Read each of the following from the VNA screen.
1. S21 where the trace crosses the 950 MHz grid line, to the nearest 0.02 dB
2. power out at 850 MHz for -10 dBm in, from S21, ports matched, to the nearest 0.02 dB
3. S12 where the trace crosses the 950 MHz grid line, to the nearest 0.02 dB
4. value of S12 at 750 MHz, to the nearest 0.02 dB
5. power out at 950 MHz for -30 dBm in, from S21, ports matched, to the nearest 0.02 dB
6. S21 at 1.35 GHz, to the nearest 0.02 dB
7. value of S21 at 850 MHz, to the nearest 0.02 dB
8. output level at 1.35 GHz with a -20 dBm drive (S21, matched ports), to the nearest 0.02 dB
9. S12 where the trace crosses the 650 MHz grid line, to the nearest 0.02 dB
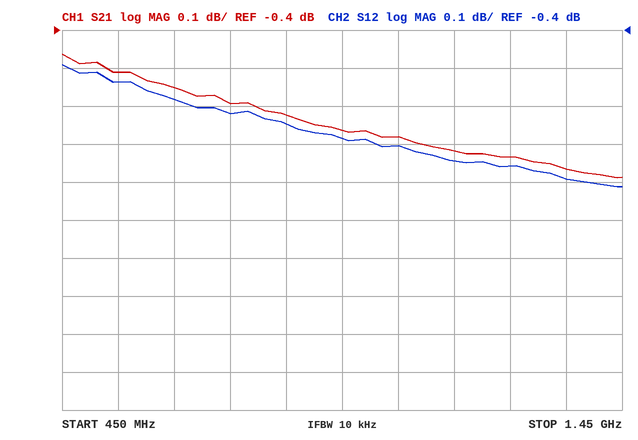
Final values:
-0.66 dB
-10.62 dBm
-0.68 dB
-0.62 dB
-30.66 dBm
-0.76 dB
-0.62 dB
-20.76 dBm
-0.58 dB
